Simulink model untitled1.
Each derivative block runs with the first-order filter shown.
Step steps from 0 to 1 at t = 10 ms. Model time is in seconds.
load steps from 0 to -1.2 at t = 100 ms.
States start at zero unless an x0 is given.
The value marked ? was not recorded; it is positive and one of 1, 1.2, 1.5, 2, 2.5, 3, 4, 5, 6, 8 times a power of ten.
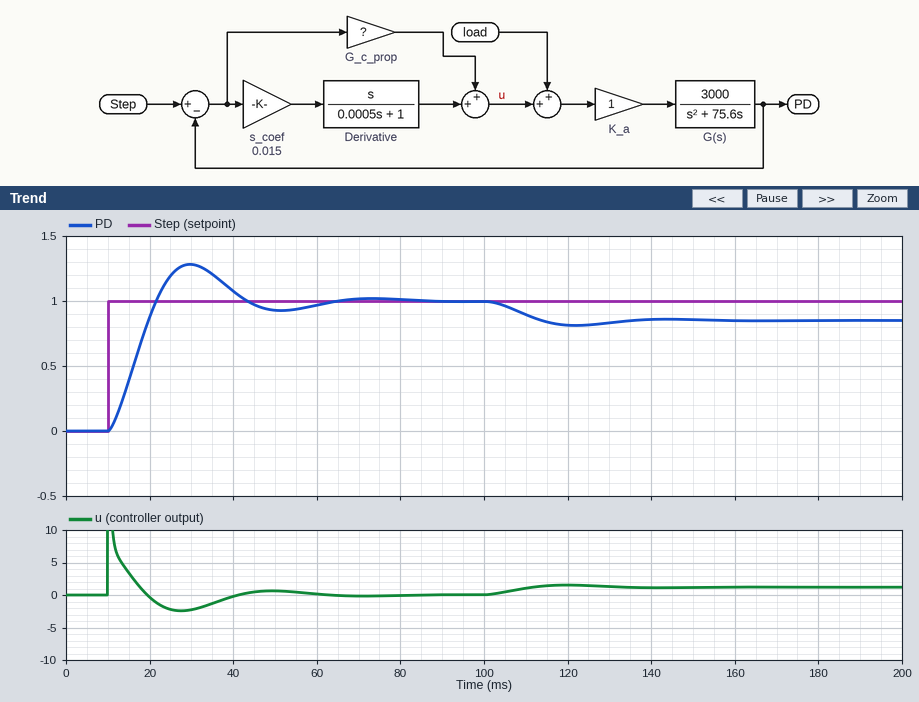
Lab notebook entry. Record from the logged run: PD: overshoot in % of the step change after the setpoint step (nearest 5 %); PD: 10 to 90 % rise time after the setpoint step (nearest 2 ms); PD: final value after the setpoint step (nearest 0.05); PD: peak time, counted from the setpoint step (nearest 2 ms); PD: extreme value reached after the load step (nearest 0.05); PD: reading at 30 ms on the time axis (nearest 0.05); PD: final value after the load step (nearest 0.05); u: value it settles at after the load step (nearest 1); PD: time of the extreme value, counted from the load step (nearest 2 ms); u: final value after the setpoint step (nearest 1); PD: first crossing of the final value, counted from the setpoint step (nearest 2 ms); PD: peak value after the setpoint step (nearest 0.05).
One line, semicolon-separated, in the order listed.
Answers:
30 %; 8 ms; 1.00; 20 ms; 0.80; 1.30; 0.85; 1; 22 ms; 0; 12 ms; 1.30
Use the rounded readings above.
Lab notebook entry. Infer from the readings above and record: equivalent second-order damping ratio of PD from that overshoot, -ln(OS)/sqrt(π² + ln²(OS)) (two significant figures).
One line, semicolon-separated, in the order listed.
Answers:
0.36
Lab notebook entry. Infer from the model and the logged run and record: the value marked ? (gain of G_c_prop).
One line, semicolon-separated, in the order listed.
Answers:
8
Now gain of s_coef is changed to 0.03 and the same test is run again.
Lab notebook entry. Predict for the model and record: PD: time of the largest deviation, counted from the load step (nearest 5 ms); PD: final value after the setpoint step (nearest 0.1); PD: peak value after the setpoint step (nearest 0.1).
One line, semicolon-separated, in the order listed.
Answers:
25 ms; 1.0; 1.2
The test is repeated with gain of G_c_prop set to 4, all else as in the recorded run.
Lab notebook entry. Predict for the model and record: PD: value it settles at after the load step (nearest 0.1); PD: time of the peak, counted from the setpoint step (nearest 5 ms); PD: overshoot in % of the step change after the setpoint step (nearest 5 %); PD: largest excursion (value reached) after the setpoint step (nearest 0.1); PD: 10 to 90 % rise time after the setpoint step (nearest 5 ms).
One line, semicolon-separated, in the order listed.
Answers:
0.7; 30 ms; 15 %; 1.1; 15 ms
